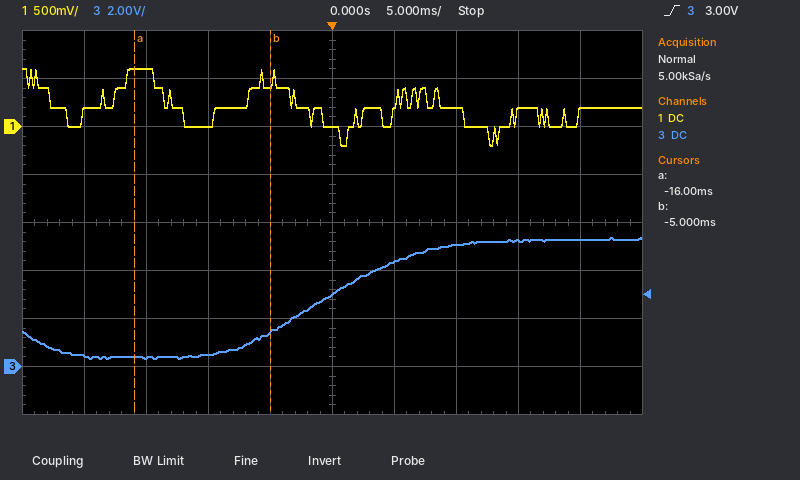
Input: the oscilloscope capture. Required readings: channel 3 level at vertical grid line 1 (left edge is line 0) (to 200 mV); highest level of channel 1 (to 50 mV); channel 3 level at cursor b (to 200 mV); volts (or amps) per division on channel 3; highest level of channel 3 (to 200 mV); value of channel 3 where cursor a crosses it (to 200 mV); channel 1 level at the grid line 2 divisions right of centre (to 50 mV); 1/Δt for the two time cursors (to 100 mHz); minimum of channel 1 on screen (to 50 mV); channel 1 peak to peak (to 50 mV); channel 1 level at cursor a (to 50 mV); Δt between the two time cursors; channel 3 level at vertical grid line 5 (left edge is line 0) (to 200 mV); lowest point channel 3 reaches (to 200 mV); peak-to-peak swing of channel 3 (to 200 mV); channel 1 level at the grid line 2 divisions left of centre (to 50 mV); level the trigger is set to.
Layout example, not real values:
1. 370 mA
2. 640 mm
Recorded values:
1. 400 mV
2. 600 mV
3. 1.4 V
4. 2 V
5. 5.4 V
6. 400 mV
7. 200 mV
8. 90.9 Hz
9. -200 mV
10. 800 mV
11. 600 mV
12. 11.0 ms
13. 3.0 V
14. 400 mV
15. 5.0 V
16. 0 mV
17. 3.00 V
